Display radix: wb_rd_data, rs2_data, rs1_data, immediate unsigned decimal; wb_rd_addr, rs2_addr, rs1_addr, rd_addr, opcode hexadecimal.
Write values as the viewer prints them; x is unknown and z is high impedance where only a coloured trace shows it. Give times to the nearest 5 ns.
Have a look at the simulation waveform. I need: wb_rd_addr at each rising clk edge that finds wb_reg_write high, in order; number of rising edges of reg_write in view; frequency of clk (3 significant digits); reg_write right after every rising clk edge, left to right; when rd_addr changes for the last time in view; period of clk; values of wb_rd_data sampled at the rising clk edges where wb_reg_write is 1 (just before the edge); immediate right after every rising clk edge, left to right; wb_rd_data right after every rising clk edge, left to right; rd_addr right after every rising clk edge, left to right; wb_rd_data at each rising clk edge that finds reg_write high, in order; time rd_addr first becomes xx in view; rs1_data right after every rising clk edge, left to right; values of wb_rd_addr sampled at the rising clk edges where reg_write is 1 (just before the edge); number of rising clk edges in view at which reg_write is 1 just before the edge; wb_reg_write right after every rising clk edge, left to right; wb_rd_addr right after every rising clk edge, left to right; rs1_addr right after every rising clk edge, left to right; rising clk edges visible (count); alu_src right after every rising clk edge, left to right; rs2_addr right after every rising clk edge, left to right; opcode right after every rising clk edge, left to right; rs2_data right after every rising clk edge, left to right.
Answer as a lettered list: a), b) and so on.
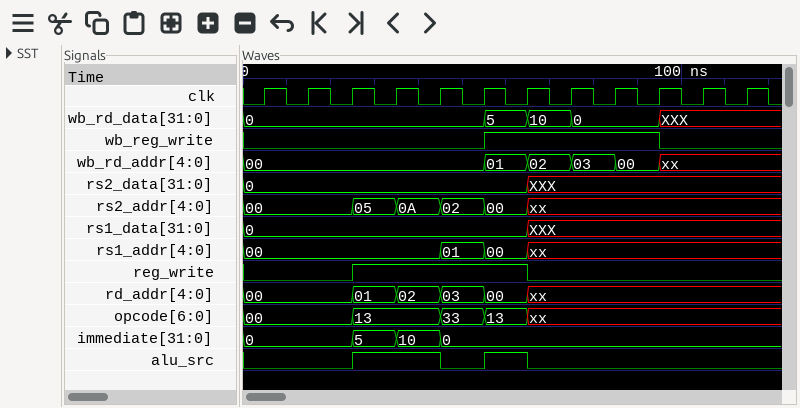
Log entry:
a) 01, 02, 03, 00
b) 1
c) 100 MHz
d) 0 0 1 1 1 1 0 0 0 0 0 0
e) 65 ns
f) 10 ns
g) 5, 10, 0, 0
h) 0, 0, 5, 10, 0, 0, 0, 0, 0, 0, 0, 0
i) 0, 0, 0, 0, 0, 5, 10, 0, 0, XXX, XXX, XXX
j) 00, 00, 01, 02, 03, 00, xx, xx, xx, xx, xx, xx
k) 0, 0, 0, 5
l) 65 ns
m) 0, 0, 0, 0, 0, 0, XXX, XXX, XXX, XXX, XXX, XXX
n) 00, 00, 00, 01
o) 4
p) 0 0 0 0 0 1 1 1 1 0 0 0
q) 00, 00, 00, 00, 00, 01, 02, 03, 00, xx, xx, xx
r) 00, 00, 00, 00, 01, 00, xx, xx, xx, xx, xx, xx
s) 12
t) 0 0 1 1 0 1 0 0 0 0 0 0
u) 00, 00, 05, 0A, 02, 00, xx, xx, xx, xx, xx, xx
v) 00, 00, 13, 13, 33, 13, xx, xx, xx, xx, xx, xx
w) 0, 0, 0, 0, 0, 0, XXX, XXX, XXX, XXX, XXX, XXX
